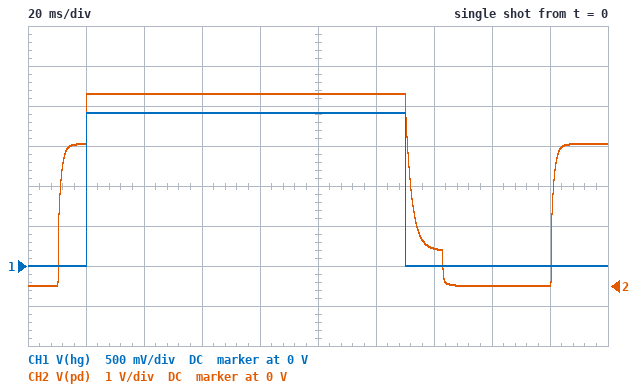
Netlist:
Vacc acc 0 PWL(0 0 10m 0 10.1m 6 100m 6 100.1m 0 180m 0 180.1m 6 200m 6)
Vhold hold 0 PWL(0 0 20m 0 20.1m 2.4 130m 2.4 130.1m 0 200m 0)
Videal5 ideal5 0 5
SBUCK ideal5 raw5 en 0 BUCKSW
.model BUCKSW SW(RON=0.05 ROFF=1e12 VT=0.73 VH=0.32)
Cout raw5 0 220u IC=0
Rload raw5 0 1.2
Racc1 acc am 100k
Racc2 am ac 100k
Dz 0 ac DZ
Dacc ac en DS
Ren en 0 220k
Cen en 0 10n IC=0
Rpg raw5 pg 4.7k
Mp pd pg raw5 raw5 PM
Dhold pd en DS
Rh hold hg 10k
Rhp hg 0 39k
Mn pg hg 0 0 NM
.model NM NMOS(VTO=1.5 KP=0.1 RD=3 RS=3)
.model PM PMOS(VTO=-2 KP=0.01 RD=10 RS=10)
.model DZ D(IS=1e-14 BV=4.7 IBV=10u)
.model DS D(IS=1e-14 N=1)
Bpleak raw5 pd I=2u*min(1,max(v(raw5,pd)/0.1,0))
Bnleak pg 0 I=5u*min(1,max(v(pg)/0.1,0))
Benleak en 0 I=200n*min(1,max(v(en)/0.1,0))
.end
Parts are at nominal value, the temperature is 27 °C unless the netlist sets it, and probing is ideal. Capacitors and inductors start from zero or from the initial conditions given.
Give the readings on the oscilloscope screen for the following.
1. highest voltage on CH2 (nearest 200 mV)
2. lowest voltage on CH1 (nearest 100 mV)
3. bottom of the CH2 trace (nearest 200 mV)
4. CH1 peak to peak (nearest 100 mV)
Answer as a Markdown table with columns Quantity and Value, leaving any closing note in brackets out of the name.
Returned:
| Quantity | Value |
|---|---|
| highest voltage on CH2 | 4.8 V |
| lowest voltage on CH1 | 0 V |
| bottom of the CH2 trace | 0 V |
| CH1 peak to peak | 1.9 V |
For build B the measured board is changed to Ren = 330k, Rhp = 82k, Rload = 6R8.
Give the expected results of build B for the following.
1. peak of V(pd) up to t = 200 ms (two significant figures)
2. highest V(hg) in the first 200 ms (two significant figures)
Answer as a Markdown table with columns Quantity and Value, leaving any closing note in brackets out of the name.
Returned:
| Quantity | Value |
|---|---|
| peak of V(pd) up to t = 200 ms | 5.0 V |
| highest V(hg) in the first 200 ms | 2.1 V |
